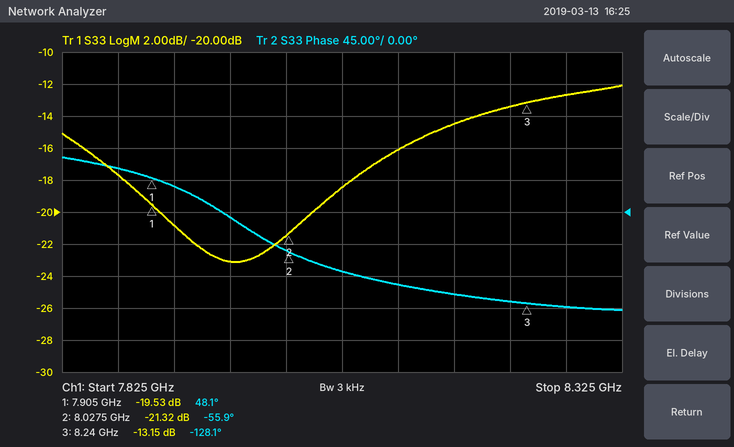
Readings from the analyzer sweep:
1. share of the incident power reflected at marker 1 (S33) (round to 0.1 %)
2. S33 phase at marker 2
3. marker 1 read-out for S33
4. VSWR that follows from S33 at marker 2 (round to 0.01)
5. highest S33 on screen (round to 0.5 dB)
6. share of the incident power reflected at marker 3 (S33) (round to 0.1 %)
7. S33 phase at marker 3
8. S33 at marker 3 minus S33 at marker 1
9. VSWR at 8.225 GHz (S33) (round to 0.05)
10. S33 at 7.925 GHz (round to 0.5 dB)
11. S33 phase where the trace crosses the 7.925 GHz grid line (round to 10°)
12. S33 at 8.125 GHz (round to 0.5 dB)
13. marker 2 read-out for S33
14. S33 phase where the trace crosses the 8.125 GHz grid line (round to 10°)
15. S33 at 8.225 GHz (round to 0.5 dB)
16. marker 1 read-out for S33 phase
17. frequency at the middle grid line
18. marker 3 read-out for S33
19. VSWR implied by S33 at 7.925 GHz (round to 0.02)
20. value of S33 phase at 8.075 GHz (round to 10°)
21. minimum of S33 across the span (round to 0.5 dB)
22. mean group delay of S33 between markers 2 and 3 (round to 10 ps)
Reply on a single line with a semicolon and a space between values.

1.1 %; -55.9°; -19.53 dB; 1.19; -12.0 dB; 4.8 %; -128.1°; 6.38 dB; 1.55; -21.0 dB; 40°; -16.0 dB; -21.32 dB; -100°; -13.5 dB; 48.1°; 8.075 GHz; -13.15 dB; 1.20; -80°; -23.0 dB; 940 ps
